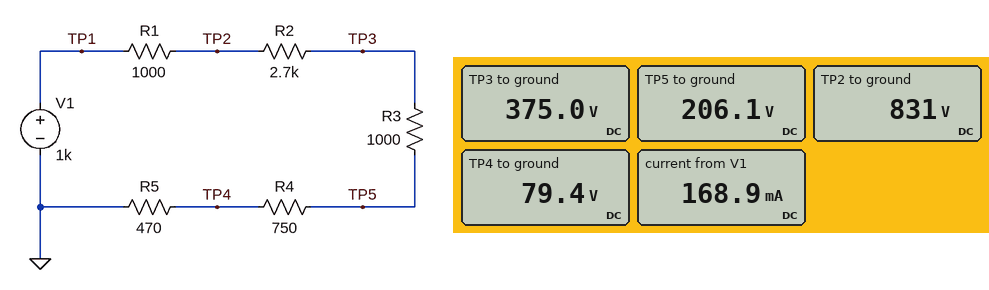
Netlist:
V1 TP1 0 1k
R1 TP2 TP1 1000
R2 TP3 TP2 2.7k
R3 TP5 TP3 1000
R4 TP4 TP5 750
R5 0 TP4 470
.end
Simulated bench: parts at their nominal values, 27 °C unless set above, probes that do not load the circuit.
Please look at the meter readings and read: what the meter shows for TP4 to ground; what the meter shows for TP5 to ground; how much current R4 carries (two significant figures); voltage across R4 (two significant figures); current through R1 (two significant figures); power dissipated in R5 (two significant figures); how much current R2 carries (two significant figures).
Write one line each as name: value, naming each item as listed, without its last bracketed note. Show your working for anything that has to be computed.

what the meter shows for TP4 to ground: 79.4 V
what the meter shows for TP5 to ground: 206.1 V
how much current R4 carries: (206.1 V - 79.4 V) / 750 Ω = 170 mA
voltage across R4: 206.1 V - 79.4 V = 130 V
current through R1: (1 kV - 831 V) / 1 kΩ = 170 mA
power dissipated in R5: (79.4 V)^2 / 470 Ω = 13 W
how much current R2 carries: (831 V - 375 V) / 2.7 kΩ = 170 mA
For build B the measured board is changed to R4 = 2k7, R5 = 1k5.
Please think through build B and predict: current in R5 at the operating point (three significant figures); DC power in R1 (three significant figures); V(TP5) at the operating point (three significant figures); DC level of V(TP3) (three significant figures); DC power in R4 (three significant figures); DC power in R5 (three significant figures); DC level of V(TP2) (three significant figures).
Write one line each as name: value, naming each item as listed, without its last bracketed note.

current in R5 at the operating point: 112 mA
DC power in R1: 12.6 W
V(TP5) at the operating point: 472 V
DC level of V(TP3): 584 V
DC power in R4: 34.1 W
DC power in R5: 18.9 W
DC level of V(TP2): 888 V
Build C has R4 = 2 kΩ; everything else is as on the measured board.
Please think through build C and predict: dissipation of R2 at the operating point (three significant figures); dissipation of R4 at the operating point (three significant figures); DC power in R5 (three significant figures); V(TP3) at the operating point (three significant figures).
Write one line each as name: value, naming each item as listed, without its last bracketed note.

dissipation of R2 at the operating point: 52.5 W
dissipation of R4 at the operating point: 38.9 W
DC power in R5: 9.14 W
V(TP3) at the operating point: 484 V
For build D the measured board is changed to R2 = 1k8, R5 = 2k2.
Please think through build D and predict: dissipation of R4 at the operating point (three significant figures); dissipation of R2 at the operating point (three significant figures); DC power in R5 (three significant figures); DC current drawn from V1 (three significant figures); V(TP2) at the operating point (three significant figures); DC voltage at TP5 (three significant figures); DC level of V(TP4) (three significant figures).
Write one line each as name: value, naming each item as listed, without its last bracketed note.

dissipation of R4 at the operating point: 16.5 W
dissipation of R2 at the operating point: 39.5 W
DC power in R5: 48.3 W
DC current drawn from V1: 148 mA
V(TP2) at the operating point: 852 V
DC voltage at TP5: 437 V
DC level of V(TP4): 326 V
